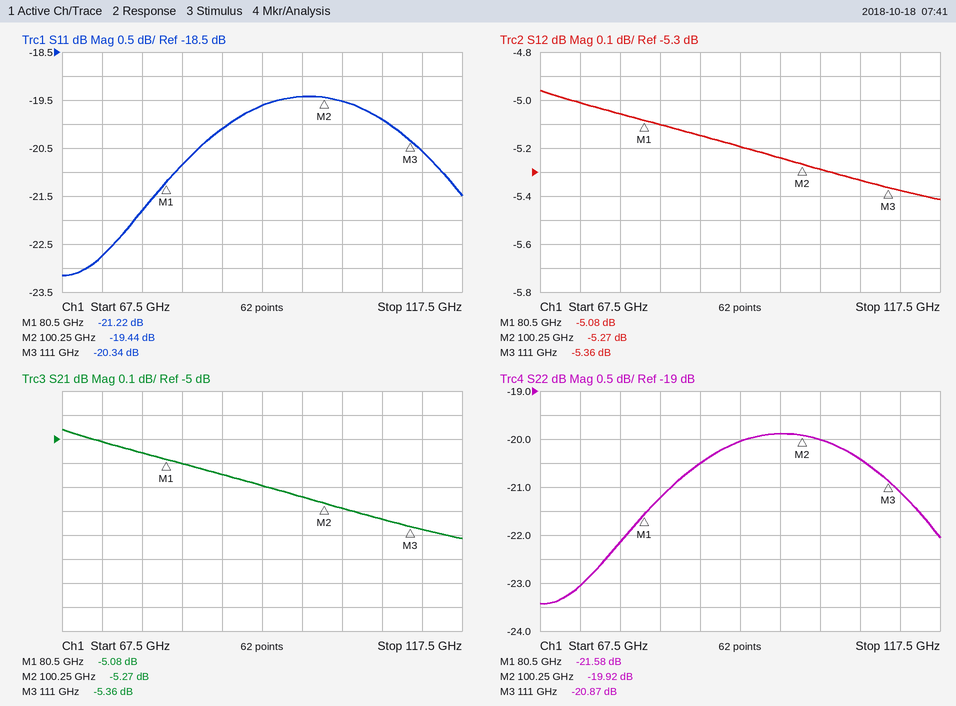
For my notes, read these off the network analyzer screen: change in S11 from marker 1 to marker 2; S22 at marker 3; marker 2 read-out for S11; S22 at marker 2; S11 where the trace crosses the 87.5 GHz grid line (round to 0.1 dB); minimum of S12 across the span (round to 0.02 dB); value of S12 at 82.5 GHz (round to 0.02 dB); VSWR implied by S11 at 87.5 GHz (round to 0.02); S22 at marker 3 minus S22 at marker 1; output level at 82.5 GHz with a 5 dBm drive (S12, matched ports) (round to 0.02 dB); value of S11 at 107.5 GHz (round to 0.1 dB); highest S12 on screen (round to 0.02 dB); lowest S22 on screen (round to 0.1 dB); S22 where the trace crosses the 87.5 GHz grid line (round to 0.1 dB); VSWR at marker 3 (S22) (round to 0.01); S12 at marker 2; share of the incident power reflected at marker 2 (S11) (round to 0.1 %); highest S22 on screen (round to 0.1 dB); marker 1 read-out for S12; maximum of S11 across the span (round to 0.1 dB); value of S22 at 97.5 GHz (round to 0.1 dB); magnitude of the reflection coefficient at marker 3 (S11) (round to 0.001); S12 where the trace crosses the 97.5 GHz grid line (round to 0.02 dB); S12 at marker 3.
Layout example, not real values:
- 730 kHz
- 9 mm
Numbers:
- 1.78 dB
- -20.87 dB
- -19.44 dB
- -19.92 dB
- -20.1 dB
- -5.42 dB
- -5.10 dB
- 1.22
- 0.71 dB
- -0.10 dBm
- -19.9 dB
- -4.96 dB
- -23.4 dB
- -20.5 dB
- 1.20
- -5.27 dB
- 1.1 %
- -19.9 dB
- -5.08 dB
- -19.4 dB
- -19.9 dB
- 0.096
- -5.24 dB
- -5.36 dB
